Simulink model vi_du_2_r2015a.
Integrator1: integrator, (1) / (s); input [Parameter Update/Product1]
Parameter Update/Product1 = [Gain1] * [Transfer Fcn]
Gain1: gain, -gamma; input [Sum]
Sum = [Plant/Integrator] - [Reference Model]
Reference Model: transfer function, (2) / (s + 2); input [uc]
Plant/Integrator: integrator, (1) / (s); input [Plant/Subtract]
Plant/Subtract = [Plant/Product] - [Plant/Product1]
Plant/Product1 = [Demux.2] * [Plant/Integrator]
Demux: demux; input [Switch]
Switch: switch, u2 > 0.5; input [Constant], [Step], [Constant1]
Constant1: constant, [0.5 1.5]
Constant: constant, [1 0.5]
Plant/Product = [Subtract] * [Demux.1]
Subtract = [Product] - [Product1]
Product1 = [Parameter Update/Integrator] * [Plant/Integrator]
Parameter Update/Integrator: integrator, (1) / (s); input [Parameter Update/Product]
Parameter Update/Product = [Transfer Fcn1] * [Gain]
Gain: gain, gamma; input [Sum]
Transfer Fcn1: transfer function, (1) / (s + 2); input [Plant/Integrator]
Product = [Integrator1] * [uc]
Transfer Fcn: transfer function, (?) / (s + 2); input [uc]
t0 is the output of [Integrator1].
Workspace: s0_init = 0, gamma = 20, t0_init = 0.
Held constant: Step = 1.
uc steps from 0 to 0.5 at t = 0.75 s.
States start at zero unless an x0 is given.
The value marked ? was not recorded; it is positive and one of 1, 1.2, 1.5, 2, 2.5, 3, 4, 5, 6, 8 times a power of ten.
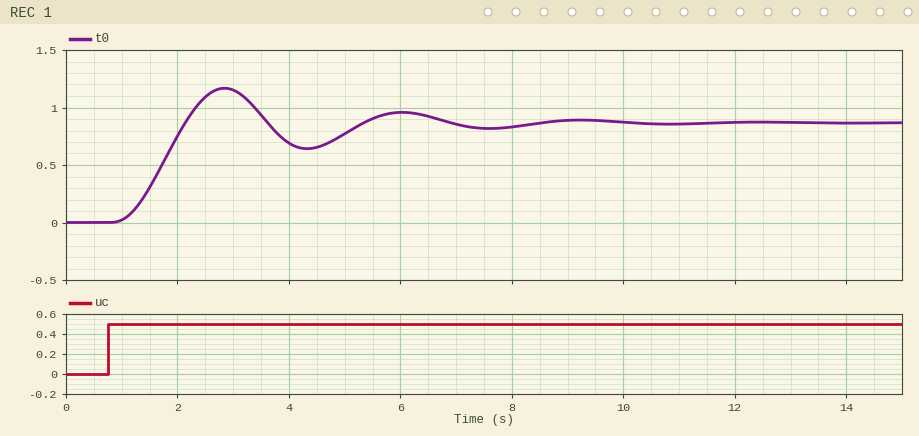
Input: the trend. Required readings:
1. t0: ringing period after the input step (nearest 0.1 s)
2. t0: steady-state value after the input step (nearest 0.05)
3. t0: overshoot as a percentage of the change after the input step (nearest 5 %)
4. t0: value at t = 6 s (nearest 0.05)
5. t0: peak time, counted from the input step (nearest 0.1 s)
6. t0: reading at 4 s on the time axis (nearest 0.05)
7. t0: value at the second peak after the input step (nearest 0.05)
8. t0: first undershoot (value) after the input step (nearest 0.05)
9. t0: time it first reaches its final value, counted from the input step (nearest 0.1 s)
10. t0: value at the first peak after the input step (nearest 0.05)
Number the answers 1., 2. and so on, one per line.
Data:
1. 3.2 s
2. 0.85
3. 35 %
4. 0.95
5. 2.1 s
6. 0.70
7. 0.95
8. 0.65
9. 1.4 s
10. 1.15
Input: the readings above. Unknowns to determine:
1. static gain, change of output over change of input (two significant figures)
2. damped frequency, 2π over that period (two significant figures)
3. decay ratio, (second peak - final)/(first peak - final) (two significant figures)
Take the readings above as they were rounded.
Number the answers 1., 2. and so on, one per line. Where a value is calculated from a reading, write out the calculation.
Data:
1. (0.85 - 0) / (0.5 - 0) = 1.7
2. 2π / 3.2 = 2.0 rad/s
3. (0.95 - 0.85) / (1.15 - 0.85) = 0.33
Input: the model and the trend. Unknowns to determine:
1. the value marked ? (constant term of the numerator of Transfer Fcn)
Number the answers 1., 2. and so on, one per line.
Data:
1. 0.6
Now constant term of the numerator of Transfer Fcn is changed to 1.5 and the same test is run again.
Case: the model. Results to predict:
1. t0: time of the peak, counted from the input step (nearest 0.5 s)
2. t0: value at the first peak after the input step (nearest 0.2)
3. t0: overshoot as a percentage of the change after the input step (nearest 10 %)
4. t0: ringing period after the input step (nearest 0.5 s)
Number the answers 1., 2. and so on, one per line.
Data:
1. 1.5 s
2. 1.6
3. 80 %
4. 2.5 s
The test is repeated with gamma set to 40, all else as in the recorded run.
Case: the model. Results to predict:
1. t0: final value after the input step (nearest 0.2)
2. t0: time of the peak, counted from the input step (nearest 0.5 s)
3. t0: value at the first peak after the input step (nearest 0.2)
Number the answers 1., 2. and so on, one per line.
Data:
1. 1.0
2. 1.5 s
3. 1.4
